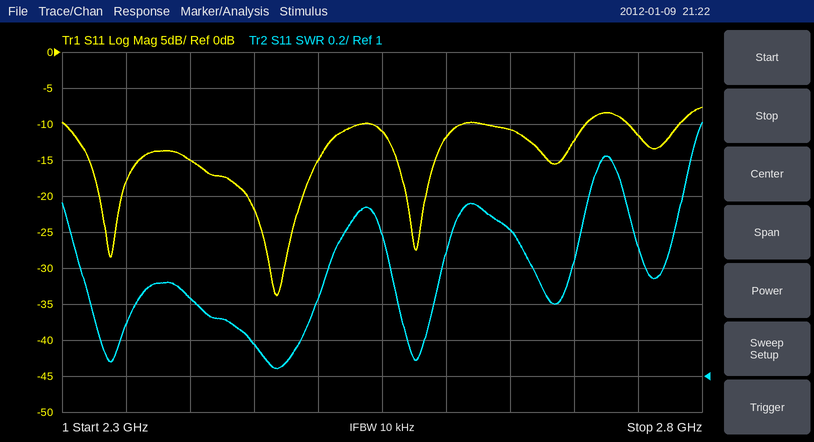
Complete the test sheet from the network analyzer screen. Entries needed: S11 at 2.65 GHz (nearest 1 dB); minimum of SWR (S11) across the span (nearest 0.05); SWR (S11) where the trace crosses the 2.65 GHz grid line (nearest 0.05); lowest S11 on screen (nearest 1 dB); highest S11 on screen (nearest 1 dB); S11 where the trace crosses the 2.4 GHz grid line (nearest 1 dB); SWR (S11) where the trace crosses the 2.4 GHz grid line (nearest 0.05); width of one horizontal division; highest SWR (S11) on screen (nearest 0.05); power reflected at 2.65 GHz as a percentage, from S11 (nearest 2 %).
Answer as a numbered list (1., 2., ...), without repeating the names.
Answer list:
1. -11 dB
2. 1.05
3. 1.80
4. -34 dB
5. -8 dB
6. -15 dB
7. 1.45
8. 50 MHz
9. 2.40
10. 8 %
